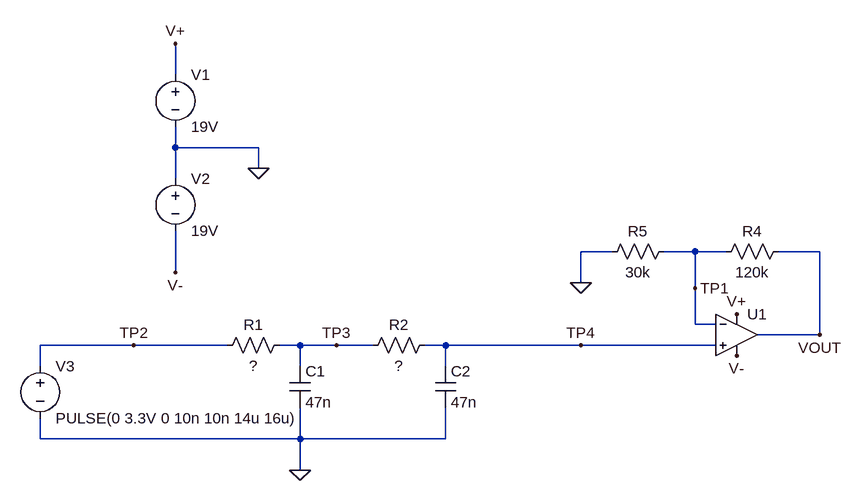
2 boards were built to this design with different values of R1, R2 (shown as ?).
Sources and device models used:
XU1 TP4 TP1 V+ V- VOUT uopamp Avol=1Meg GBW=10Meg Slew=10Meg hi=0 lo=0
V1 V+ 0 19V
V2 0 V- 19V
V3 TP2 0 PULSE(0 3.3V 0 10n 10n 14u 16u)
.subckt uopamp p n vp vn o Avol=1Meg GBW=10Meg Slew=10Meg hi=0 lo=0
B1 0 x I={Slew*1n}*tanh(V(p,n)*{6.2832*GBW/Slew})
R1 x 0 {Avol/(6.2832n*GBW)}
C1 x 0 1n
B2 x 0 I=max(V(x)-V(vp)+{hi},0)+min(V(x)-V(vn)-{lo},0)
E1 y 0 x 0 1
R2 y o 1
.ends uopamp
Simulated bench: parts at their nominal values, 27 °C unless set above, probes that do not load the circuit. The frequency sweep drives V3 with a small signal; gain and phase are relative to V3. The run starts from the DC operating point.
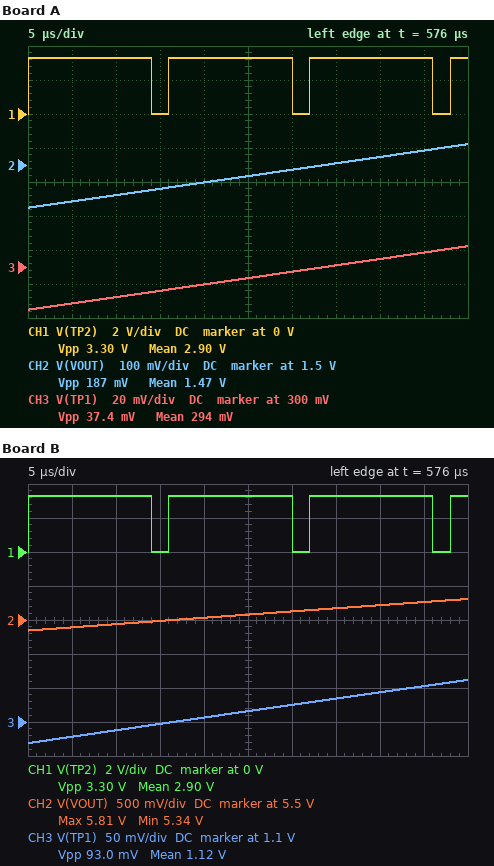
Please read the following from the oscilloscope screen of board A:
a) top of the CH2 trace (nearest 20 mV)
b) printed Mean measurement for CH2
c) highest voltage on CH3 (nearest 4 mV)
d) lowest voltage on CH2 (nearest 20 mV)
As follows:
1.56 V
1.47 V
312 mV
1.38 V
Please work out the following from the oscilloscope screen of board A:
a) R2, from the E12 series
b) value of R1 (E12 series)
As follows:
27 kΩ
18 kΩ
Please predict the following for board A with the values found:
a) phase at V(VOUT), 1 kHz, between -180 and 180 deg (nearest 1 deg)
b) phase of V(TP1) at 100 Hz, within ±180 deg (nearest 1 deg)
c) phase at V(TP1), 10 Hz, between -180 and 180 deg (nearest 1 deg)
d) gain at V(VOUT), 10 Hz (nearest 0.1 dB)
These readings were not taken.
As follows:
-156 deg
-73 deg
-11 deg
13.9 dB
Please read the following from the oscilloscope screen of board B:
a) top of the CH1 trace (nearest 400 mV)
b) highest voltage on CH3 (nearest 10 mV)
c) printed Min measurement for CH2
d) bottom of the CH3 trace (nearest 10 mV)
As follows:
3.2 V
1.16 V
5.34 V
1.07 V
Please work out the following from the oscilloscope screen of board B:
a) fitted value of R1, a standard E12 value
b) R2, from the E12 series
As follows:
3.9 kΩ
15 kΩ
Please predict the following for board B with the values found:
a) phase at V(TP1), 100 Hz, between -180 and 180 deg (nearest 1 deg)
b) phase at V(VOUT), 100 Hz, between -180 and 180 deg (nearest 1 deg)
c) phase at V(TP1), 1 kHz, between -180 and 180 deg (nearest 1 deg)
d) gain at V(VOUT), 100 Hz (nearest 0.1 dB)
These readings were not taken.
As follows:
-35 deg
-35 deg
-121 deg
12.7 dB
